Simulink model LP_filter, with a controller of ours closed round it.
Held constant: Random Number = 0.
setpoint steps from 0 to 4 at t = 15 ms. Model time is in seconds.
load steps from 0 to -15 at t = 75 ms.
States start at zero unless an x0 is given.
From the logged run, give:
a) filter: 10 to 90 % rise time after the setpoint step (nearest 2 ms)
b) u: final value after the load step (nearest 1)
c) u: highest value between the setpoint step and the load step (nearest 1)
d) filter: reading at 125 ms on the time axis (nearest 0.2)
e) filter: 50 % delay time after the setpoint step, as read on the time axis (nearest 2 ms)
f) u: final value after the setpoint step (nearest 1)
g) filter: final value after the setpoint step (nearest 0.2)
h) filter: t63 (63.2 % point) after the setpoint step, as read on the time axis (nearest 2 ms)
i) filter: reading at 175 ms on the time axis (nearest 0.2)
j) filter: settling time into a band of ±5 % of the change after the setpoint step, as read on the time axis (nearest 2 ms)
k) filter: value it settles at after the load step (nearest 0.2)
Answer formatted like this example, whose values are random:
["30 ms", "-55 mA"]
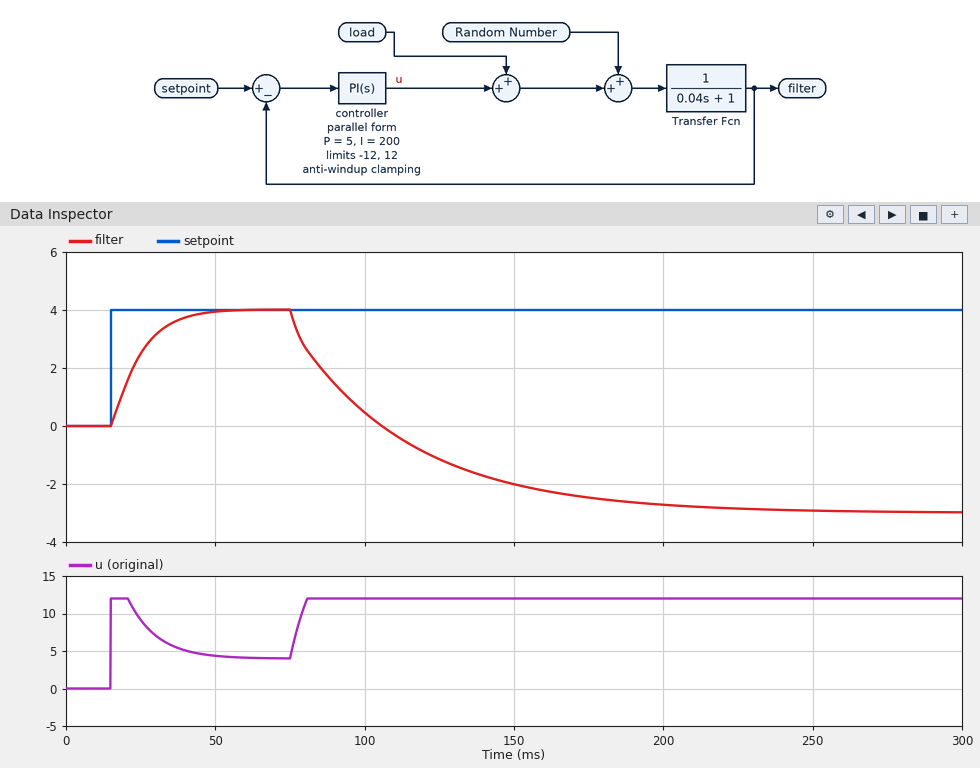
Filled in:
["20 ms", "12", "12", "-1.2", "22 ms", "4", "4.0", "26 ms", "-2.4", "42 ms", "-3.0"]
